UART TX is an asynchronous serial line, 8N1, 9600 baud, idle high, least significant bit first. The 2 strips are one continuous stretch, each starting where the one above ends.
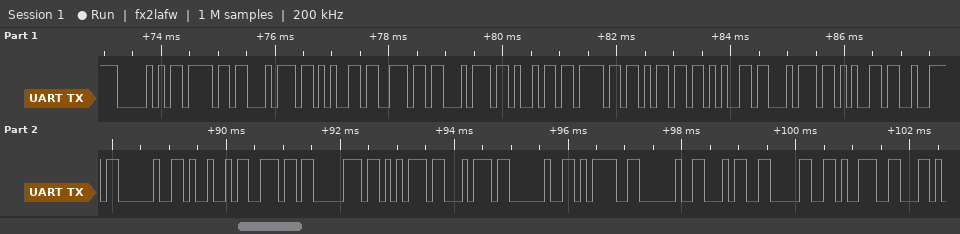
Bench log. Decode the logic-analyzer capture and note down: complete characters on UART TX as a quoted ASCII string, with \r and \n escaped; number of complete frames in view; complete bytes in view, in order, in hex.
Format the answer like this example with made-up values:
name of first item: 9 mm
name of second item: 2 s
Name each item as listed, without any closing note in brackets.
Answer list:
complete characters on UART TX as a quoted ASCII string, with \r and \n escaped: "Potentiometer Input = 409"
number of complete frames in view: 25
complete bytes in view, in order, in hex: 50 6F 74 65 6E 74 69 6F 6D 65 74 65 72 20 49 6E 70 75 74 20 3D 20 34 30 39
